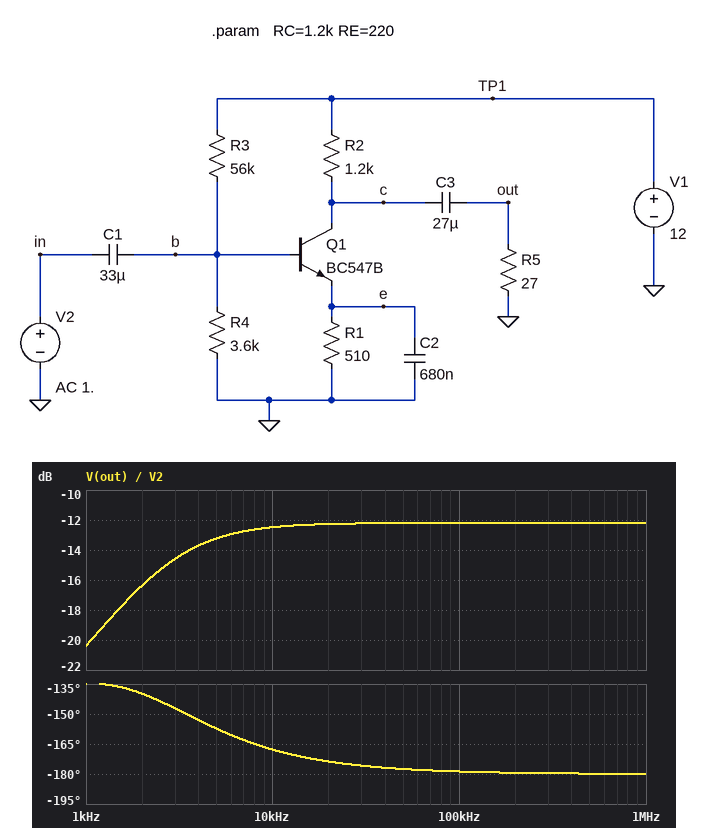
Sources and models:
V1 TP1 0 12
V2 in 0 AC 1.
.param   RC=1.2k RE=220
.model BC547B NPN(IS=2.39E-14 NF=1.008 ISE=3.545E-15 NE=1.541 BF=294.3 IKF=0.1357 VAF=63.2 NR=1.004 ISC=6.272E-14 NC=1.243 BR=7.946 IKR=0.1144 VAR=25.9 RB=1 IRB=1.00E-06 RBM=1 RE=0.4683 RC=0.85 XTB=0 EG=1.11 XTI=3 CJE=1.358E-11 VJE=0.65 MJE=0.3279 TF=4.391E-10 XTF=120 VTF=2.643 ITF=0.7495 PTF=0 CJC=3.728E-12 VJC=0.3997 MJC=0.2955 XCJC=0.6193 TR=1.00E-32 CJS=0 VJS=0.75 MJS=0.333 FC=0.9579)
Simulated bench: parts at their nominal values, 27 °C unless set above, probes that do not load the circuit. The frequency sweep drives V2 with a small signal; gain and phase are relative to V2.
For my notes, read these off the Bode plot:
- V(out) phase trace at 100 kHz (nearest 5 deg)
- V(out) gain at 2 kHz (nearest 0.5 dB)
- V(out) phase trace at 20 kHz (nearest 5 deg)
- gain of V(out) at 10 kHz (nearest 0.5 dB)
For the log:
-180 deg
-16.5 dB
-175 deg
-12.5 dB
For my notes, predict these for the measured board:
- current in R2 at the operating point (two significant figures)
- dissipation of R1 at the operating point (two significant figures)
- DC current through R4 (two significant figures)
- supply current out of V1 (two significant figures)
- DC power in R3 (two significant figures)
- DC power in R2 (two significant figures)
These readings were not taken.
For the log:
240 µA
31 µW
200 µA
450 µA
2.3 mW
72 µW
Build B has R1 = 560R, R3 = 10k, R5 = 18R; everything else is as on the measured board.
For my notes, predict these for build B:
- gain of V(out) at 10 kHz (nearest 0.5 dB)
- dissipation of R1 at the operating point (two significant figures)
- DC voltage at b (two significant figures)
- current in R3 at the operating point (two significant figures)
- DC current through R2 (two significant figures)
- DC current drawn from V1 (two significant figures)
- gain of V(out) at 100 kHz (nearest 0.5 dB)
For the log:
-3.0 dB
11 mW
3.1 V
890 µA
4.4 mA
5.3 mA
8.0 dB
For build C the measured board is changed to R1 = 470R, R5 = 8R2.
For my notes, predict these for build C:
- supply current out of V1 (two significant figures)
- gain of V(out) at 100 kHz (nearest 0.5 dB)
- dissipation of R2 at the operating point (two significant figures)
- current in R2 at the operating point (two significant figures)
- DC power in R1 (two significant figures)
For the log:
460 µA
-22.0 dB
82 µW
260 µA
32 µW
